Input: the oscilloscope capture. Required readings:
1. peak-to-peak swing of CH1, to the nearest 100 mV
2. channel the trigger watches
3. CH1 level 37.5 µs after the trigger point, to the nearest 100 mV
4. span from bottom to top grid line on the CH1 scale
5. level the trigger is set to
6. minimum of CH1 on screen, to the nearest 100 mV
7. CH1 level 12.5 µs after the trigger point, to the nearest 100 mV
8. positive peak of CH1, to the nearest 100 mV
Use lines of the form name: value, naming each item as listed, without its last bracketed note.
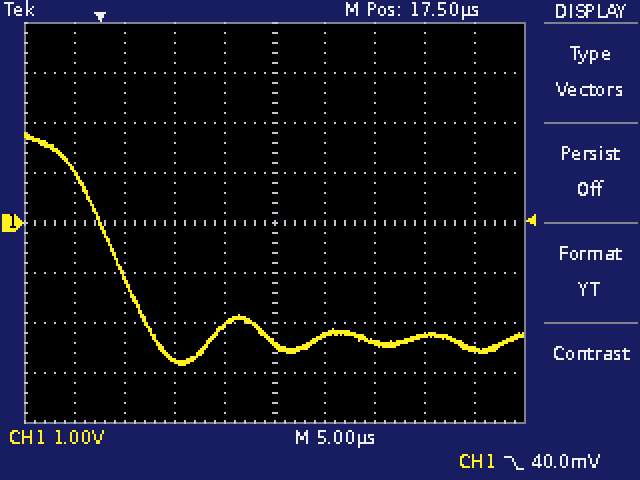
peak-to-peak swing of CH1, to the nearest 100 mV: 4.6 V
channel the trigger watches: CH1
CH1 level 37.5 µs after the trigger point, to the nearest 100 mV: -2.5 V
span from bottom to top grid line on the CH1 scale: 8 V
level the trigger is set to: 40.0 mV
minimum of CH1 on screen, to the nearest 100 mV: -2.8 V
CH1 level 12.5 µs after the trigger point, to the nearest 100 mV: -2.0 V
positive peak of CH1, to the nearest 100 mV: 1.8 V
